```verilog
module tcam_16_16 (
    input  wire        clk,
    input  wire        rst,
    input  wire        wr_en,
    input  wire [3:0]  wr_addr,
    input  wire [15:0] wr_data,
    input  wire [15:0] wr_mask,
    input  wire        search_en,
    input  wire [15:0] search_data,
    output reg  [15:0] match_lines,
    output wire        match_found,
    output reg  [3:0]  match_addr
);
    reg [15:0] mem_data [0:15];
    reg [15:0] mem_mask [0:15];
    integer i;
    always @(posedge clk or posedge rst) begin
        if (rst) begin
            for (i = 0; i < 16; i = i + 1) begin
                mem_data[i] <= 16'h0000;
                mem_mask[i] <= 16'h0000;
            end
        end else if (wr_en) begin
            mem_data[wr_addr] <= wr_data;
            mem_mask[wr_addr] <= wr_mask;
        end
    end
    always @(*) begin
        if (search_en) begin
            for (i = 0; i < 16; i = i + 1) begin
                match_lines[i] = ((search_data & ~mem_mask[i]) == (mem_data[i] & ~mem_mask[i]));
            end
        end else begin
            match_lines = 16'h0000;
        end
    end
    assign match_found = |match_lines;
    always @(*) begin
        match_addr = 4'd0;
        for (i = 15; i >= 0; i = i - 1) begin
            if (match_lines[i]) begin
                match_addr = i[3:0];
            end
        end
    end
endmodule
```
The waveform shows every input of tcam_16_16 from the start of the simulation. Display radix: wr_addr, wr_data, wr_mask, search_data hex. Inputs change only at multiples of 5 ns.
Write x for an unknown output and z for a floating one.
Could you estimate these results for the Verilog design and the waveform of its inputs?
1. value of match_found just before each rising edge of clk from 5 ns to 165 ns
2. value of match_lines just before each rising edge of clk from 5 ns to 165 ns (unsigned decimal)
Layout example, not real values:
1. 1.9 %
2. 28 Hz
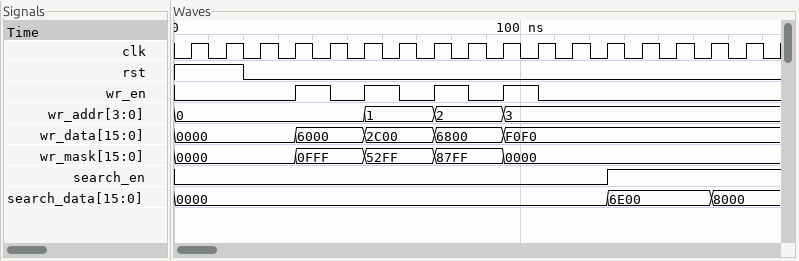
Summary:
1. 0 0 0 0 0 0 0 0 0 0 0 0 0 1 1 1 0
2. 0, 0, 0, 0, 0, 0, 0, 0, 0, 0, 0, 0, 0, 7, 7, 7, 0
